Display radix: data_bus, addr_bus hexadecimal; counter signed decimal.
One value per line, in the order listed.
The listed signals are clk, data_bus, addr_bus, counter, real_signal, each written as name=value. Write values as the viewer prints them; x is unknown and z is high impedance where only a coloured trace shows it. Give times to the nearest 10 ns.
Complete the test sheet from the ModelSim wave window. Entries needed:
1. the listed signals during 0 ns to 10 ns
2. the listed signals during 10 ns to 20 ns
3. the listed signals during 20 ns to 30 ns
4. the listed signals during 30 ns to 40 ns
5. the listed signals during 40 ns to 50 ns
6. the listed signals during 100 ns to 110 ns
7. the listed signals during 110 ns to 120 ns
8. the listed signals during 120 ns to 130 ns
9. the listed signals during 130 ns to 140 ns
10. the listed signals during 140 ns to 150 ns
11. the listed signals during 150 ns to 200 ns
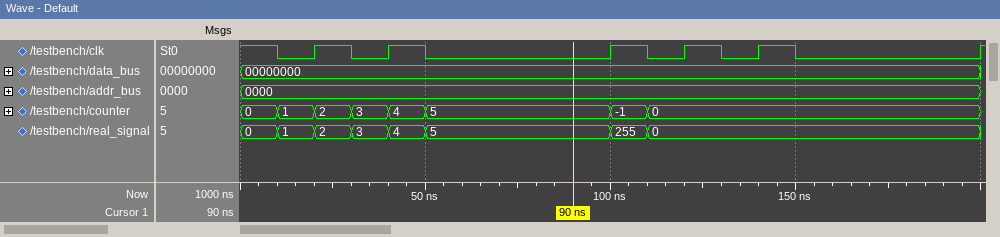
clk=1, data_bus=00000000, addr_bus=0000, counter=0, real_signal=0
clk=0, data_bus=00000000, addr_bus=0000, counter=1, real_signal=1
clk=1, data_bus=00000000, addr_bus=0000, counter=2, real_signal=2
clk=0, data_bus=00000000, addr_bus=0000, counter=3, real_signal=3
clk=1, data_bus=00000000, addr_bus=0000, counter=4, real_signal=4
clk=1, data_bus=00000000, addr_bus=0000, counter=-1, real_signal=255
clk=0, data_bus=00000000, addr_bus=0000, counter=0, real_signal=0
clk=1, data_bus=00000000, addr_bus=0000, counter=0, real_signal=0
clk=0, data_bus=00000000, addr_bus=0000, counter=0, real_signal=0
clk=1, data_bus=00000000, addr_bus=0000, counter=0, real_signal=0
clk=0, data_bus=00000000, addr_bus=0000, counter=0, real_signal=0
